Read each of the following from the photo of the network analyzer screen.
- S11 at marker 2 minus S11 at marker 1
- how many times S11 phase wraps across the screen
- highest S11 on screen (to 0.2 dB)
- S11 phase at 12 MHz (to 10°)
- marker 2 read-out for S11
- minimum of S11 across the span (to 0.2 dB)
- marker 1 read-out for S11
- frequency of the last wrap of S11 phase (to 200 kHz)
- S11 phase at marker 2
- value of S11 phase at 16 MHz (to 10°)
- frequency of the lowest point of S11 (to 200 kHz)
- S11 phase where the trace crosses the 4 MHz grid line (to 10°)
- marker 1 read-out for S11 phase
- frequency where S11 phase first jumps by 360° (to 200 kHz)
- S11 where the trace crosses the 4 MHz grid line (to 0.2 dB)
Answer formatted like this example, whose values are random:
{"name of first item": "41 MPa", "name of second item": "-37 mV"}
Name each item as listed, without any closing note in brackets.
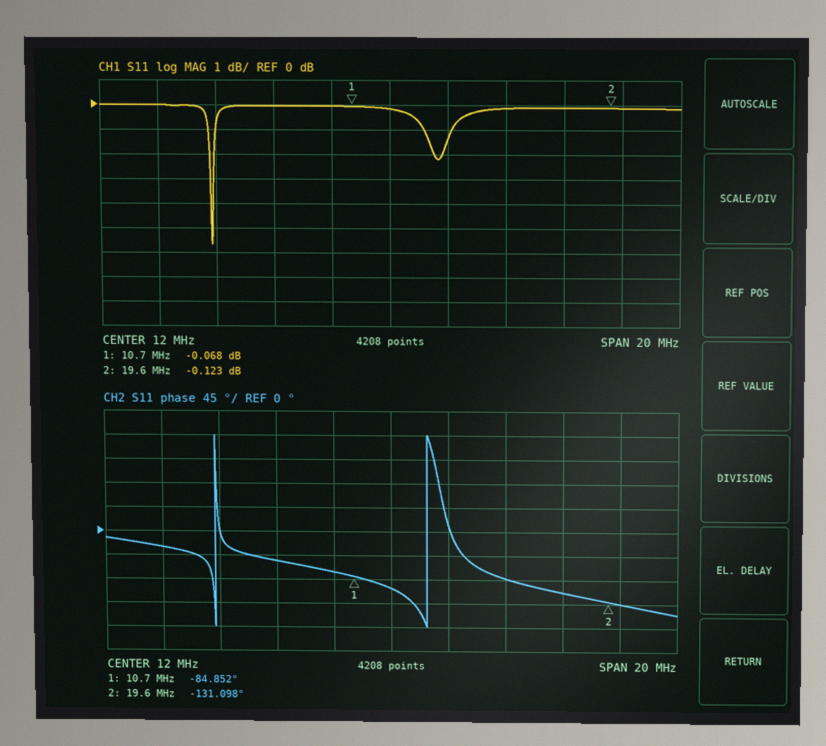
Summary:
{"S11 at marker 2 minus S11 at marker 1": "-0.055 dB", "how many times S11 phase wraps across the screen": "2", "highest S11 on screen": "0.0 dB", "S11 phase at 12 MHz": "-110°", "marker 2 read-out for S11": "-0.123 dB", "minimum of S11 across the span": "-5.6 dB", "marker 1 read-out for S11": "-0.068 dB", "frequency of the last wrap of S11 phase": "13.2 MHz", "S11 phase at marker 2": "-131.098°", "value of S11 phase at 16 MHz": "-90°", "frequency of the lowest point of S11": "5.8 MHz", "S11 phase where the trace crosses the 4 MHz grid line": "-30°", "marker 1 read-out for S11 phase": "-84.852°", "frequency where S11 phase first jumps by 360°": "5.8 MHz", "S11 where the trace crosses the 4 MHz grid line": "0.0 dB"}
